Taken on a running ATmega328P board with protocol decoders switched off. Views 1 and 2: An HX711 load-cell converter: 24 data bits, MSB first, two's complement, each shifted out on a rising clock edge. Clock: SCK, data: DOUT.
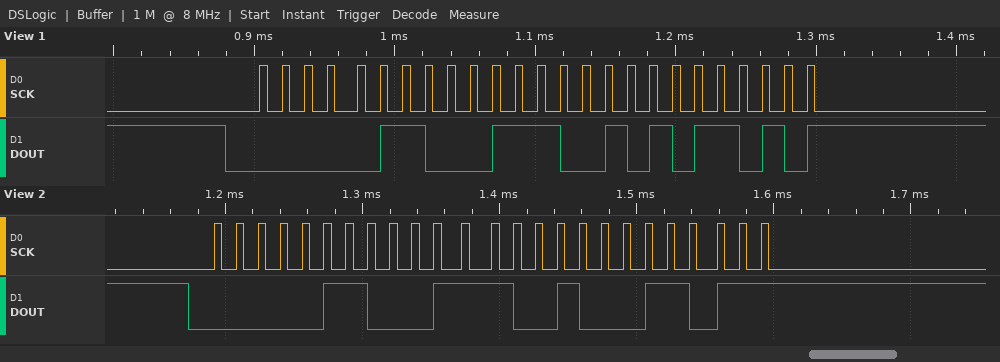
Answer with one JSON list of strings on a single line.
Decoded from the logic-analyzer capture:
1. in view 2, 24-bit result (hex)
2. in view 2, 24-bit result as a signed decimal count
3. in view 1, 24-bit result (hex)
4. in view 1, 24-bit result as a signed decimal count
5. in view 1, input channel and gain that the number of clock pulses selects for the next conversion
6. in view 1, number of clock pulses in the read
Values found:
["0x06391B", "407835", "0x06395A", "407898", "channel A, gain 128", "25"]
